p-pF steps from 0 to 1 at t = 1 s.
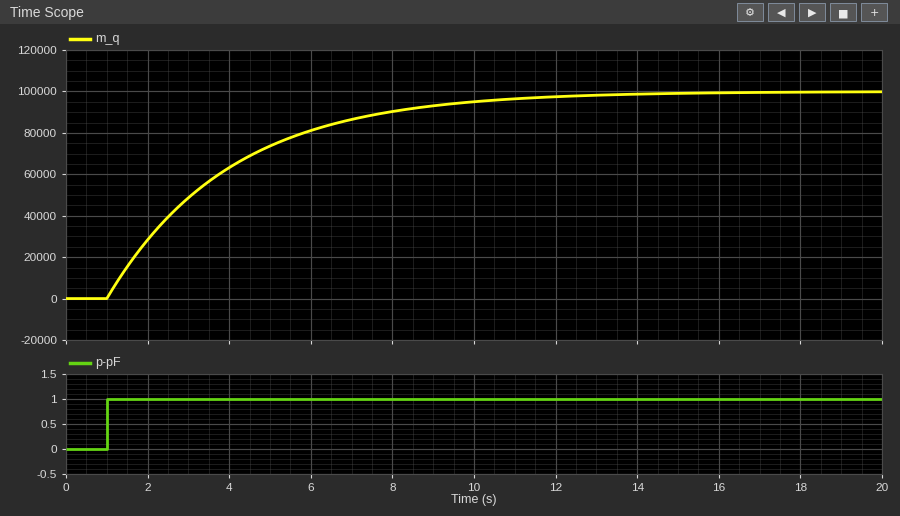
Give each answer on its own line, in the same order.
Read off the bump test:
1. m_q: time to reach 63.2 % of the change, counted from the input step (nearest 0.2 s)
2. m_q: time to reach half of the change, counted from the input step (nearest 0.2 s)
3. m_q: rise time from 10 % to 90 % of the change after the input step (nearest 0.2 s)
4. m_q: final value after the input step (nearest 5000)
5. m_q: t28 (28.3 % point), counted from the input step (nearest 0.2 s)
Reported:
3.0 s
2.0 s
6.6 s
100000
1.0 s
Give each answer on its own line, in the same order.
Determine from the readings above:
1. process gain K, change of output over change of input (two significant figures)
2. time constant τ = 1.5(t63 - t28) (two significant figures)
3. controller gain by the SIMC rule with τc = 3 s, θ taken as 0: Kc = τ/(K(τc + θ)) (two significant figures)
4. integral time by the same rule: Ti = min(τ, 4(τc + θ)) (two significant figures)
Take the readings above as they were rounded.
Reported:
100000
3.0 s
0.000010
3.0 s
